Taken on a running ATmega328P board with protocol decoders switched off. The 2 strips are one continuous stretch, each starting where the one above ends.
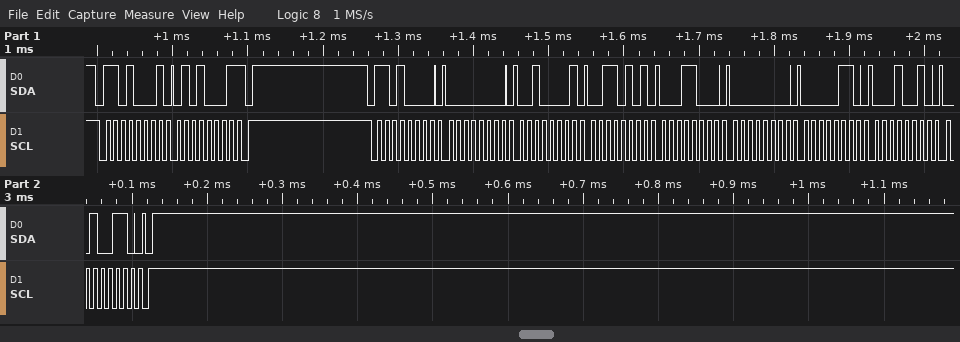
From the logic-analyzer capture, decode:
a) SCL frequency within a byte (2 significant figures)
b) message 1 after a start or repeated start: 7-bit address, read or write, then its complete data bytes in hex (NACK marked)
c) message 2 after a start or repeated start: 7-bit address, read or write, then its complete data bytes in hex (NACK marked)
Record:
100 kHz
0x68 read: 51 NACK
0x68 write: 00 21 35 18 00 06 12 26
